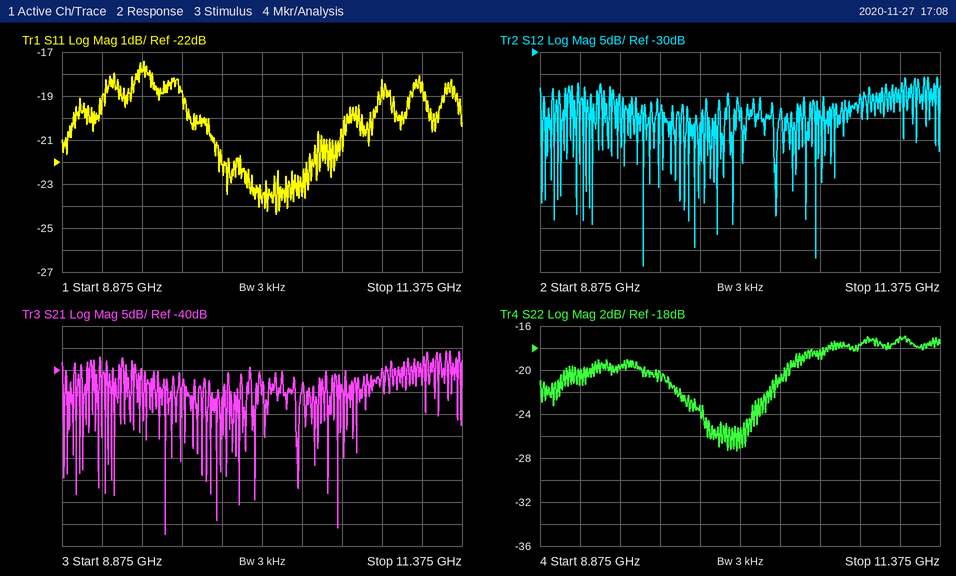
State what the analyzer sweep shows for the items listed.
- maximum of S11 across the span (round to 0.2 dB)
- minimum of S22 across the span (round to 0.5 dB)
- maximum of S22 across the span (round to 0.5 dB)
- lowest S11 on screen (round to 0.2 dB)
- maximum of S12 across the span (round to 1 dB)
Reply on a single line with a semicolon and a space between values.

-17.4 dB; -27.5 dB; -17.0 dB; -24.4 dB; -36 dB
